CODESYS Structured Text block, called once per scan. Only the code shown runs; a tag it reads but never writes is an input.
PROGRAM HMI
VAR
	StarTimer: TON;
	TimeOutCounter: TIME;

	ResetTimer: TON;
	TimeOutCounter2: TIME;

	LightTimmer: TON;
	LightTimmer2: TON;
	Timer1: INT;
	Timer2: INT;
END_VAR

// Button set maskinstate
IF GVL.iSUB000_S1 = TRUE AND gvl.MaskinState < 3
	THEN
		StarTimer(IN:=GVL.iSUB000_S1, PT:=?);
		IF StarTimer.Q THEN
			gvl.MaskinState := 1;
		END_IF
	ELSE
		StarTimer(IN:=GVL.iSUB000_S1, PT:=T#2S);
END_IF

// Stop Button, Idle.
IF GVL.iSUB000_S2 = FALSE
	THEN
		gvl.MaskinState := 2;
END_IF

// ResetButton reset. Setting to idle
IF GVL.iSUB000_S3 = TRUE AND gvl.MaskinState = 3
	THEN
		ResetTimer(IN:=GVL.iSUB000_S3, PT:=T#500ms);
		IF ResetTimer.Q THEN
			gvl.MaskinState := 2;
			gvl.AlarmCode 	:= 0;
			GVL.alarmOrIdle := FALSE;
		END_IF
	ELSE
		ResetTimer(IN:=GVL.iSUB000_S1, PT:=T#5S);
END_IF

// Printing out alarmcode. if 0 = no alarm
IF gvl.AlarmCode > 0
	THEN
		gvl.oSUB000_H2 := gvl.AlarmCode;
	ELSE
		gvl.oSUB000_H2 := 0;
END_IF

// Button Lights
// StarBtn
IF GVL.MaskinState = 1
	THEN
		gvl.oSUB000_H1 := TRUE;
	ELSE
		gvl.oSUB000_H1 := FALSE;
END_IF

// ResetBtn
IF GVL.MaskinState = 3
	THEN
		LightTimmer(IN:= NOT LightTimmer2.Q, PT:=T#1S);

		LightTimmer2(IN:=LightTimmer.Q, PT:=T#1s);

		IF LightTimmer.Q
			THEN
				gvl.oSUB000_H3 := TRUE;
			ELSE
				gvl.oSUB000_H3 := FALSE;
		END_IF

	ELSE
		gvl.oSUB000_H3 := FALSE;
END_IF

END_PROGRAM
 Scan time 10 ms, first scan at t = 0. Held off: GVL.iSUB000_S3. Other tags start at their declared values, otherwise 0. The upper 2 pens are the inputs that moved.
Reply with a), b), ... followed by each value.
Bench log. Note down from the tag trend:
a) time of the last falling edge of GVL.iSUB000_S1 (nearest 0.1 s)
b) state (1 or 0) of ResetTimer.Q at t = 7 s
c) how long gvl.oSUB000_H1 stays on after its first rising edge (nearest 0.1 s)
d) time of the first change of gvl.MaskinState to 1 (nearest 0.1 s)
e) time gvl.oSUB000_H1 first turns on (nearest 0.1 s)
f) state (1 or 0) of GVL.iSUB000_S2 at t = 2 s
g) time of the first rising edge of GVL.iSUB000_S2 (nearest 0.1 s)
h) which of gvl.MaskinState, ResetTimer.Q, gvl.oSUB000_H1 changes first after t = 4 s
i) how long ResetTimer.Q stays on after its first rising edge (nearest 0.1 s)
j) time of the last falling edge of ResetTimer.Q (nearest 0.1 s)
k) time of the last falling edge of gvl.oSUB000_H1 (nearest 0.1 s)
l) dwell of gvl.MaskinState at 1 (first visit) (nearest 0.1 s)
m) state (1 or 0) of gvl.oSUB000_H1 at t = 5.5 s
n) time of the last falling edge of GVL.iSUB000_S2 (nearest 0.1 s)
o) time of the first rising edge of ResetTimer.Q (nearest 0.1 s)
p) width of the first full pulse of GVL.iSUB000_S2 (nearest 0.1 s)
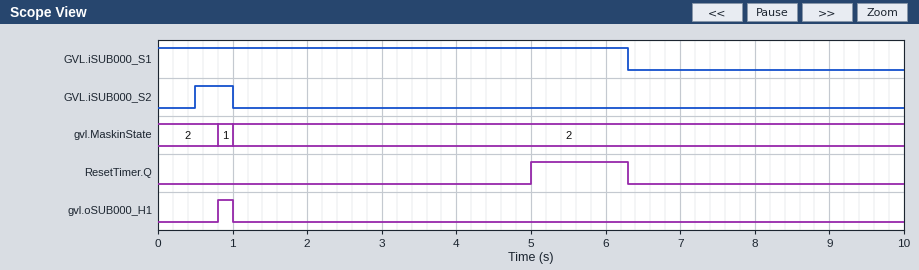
a) 6.3 s
b) 0
c) 0.2 s
d) 0.8 s
e) 0.8 s
f) 0
g) 0.5 s
h) ResetTimer.Q
i) 1.3 s
j) 6.3 s
k) 1.0 s
l) 0.2 s
m) 0
n) 1.0 s
o) 5.0 s
p) 0.5 s
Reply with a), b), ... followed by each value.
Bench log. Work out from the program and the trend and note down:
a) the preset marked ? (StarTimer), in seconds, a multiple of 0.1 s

a) 0.8 s
